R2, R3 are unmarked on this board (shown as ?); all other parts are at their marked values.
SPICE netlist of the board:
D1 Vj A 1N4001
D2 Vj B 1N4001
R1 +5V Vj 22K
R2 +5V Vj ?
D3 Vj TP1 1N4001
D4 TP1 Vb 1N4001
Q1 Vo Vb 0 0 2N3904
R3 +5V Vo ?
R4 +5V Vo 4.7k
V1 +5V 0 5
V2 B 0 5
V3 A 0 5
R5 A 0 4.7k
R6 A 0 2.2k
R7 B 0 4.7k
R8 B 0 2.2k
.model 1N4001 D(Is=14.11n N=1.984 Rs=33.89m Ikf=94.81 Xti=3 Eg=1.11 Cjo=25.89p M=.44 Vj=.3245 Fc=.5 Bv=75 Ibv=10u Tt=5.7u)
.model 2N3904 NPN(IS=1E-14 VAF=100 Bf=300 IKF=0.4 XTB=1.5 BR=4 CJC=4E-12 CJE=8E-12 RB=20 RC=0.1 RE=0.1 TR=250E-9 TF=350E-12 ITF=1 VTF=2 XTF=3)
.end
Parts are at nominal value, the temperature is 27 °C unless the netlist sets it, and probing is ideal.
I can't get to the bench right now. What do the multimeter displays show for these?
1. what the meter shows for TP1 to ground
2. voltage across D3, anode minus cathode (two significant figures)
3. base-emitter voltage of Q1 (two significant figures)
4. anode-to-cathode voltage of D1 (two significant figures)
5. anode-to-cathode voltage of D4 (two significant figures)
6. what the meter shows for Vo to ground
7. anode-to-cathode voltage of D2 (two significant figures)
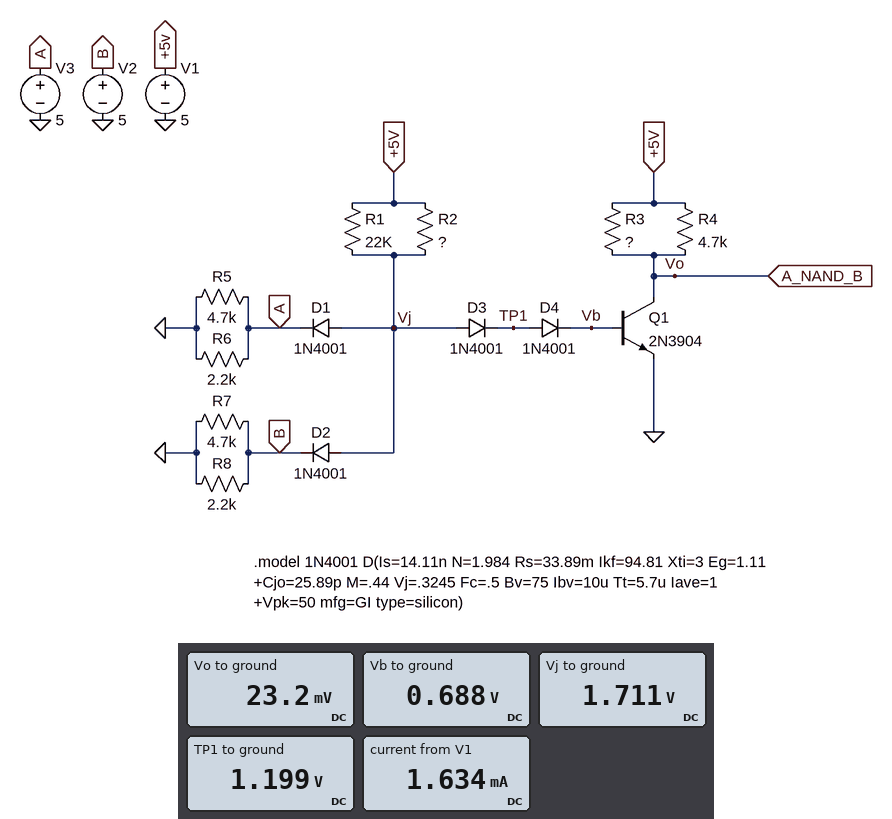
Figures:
1.199 V
510 mV
690 mV
-3.3 V
510 mV
23.2 mV
-3.3 V
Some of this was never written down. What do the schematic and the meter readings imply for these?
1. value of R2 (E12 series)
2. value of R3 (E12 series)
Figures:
22 kΩ
18 kΩ
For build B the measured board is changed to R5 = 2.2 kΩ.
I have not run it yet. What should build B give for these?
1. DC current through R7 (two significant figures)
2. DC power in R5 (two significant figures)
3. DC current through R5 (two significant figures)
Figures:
1.1 mA
11 mW
2.3 mA
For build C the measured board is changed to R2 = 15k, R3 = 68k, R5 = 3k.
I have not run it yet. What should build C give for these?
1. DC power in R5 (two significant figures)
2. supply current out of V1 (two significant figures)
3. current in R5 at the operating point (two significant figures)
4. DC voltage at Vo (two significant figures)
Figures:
8.3 mW
1.5 mA
1.7 mA
19 mV
